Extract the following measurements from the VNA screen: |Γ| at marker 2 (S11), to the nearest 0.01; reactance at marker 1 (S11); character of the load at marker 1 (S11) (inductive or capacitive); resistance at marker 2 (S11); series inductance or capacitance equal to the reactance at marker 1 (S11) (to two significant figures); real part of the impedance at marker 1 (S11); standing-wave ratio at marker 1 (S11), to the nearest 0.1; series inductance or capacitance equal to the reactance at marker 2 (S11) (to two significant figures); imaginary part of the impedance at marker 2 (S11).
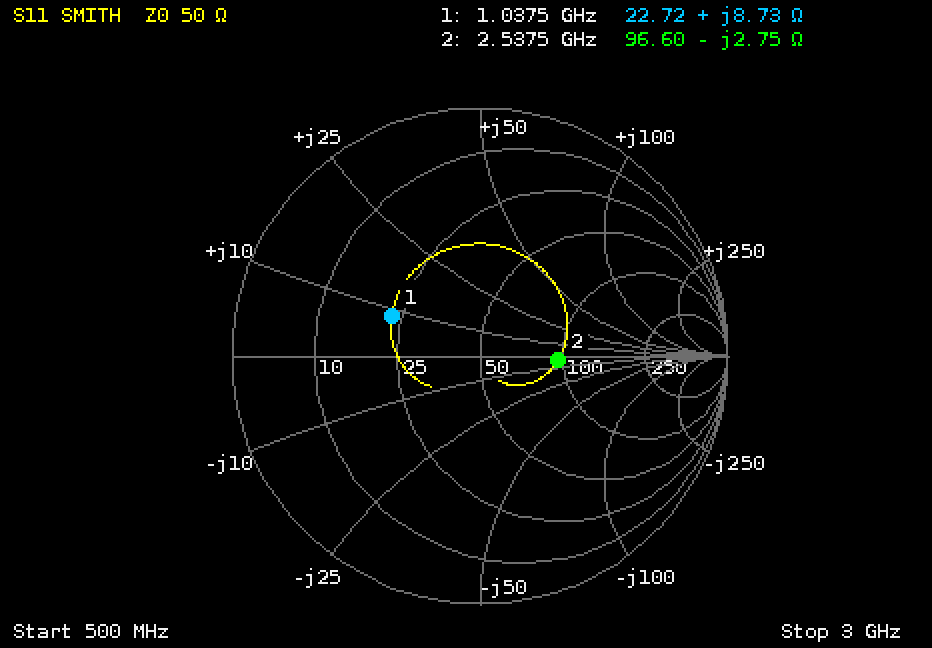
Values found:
0.32
+8.73 Ω
inductive
96.60 Ω
1.3 nH
22.72 Ω
2.3
23 pF
-2.75 Ω
